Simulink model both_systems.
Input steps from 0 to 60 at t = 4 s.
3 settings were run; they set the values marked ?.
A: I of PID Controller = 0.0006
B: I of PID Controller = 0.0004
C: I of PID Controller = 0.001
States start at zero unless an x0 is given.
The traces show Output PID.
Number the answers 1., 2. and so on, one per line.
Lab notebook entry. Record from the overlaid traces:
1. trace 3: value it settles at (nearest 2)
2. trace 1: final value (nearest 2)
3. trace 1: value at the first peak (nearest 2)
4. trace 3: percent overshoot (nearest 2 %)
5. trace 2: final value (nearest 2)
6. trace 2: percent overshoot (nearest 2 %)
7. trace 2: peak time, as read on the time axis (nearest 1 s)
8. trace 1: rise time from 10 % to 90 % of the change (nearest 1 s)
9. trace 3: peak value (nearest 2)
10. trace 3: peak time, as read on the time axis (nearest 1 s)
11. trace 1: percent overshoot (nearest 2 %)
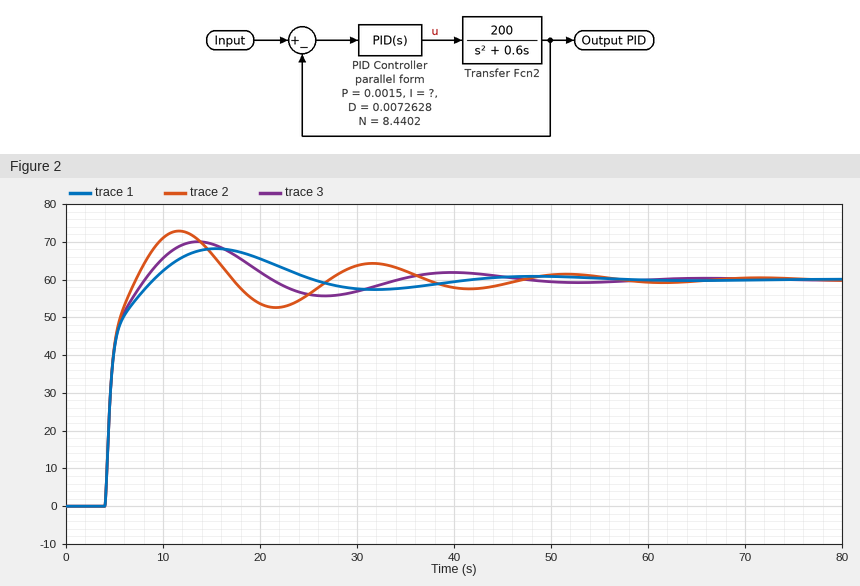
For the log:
1. 60
2. 60
3. 68
4. 16 %
5. 60
6. 22 %
7. 12 s
8. 3 s
9. 70
10. 14 s
11. 14 %
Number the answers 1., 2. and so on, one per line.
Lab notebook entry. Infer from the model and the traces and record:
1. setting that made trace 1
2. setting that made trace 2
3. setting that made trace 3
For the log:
1. B
2. C
3. A
